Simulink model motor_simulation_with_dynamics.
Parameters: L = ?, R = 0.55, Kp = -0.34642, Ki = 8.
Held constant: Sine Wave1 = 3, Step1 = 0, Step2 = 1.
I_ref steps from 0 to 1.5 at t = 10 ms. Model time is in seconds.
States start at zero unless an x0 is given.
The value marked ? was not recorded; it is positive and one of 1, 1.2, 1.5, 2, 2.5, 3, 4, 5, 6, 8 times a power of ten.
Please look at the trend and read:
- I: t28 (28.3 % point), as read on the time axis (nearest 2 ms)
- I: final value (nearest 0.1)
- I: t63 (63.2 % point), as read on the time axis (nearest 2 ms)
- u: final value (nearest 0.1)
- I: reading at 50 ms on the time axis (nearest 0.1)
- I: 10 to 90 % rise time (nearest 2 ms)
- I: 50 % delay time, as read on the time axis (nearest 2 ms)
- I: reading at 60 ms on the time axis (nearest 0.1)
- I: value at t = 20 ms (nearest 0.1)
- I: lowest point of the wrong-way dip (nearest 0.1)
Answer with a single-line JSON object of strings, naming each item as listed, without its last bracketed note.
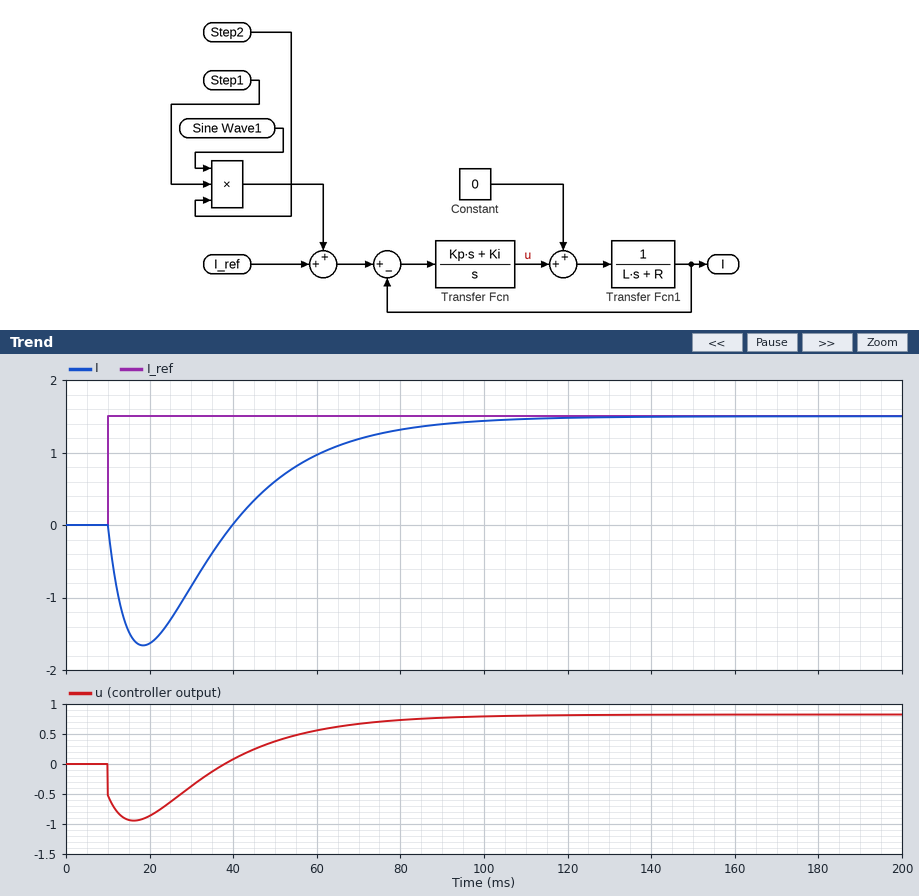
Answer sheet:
{"I: t28 (28.3 % point), as read on the time axis": "46 ms", "I: final value": "1.5", "I: t63 (63.2 % point), as read on the time axis": "60 ms", "u: final value": "0.8", "I: reading at 50 ms on the time axis": "0.6", "I: 10 to 90 % rise time": "42 ms", "I: 50 % delay time, as read on the time axis": "54 ms", "I: reading at 60 ms on the time axis": "1.0", "I: value at t = 20 ms": "-1.6", "I: lowest point of the wrong-way dip": "-1.7"}
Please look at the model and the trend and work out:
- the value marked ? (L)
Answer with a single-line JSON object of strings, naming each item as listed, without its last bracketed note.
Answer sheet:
{"the value marked ?": "0.001"}
